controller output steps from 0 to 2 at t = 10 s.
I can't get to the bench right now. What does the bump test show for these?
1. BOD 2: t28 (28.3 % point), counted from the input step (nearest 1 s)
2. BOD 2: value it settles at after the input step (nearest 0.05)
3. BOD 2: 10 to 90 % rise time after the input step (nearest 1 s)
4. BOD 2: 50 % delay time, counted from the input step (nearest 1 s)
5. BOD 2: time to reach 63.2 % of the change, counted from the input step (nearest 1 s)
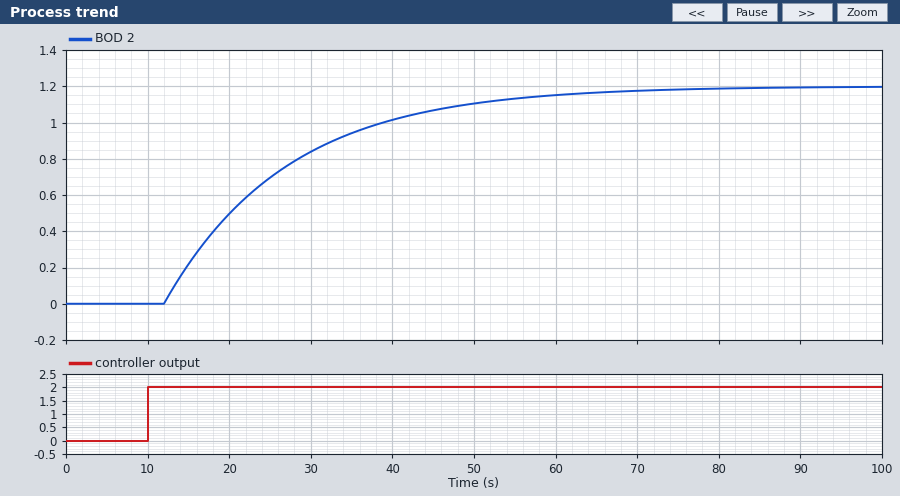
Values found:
7 s
1.20
33 s
12 s
17 s
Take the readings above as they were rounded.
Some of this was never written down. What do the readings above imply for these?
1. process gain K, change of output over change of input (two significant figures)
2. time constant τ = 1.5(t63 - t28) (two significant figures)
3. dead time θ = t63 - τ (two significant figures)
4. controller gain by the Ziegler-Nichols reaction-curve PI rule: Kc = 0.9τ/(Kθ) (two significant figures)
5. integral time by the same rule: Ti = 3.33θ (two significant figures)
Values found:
0.60
15 s
2.0 s
11
6.7 s
